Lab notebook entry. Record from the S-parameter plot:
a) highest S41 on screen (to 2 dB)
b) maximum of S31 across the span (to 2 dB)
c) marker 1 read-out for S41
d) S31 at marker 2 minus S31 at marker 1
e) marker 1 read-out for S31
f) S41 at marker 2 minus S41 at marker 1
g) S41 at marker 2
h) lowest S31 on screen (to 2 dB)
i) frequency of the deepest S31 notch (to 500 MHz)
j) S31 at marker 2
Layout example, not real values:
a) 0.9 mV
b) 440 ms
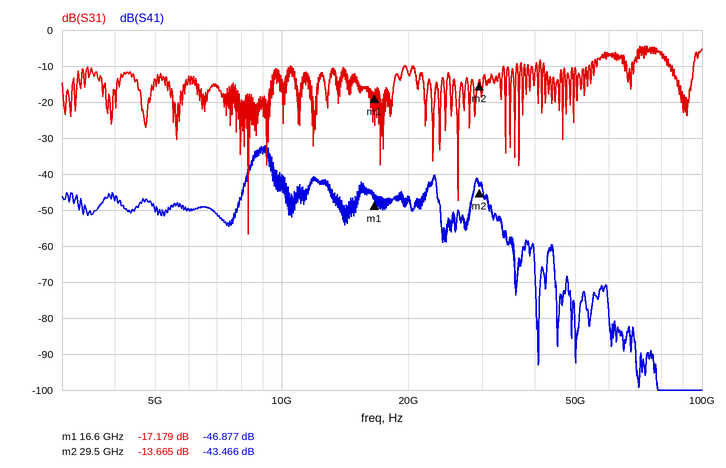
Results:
a) -32 dB
b) -4 dB
c) -46.877 dB
d) 3.514 dB
e) -17.179 dB
f) 3.411 dB
g) -43.466 dB
h) -56 dB
i) 8.5 GHz
j) -13.665 dB
